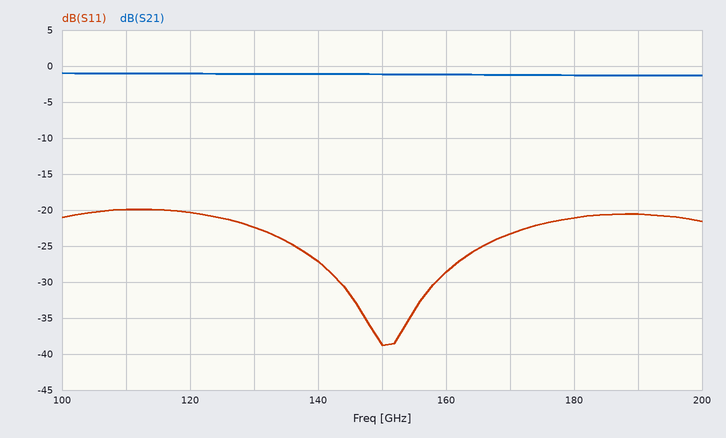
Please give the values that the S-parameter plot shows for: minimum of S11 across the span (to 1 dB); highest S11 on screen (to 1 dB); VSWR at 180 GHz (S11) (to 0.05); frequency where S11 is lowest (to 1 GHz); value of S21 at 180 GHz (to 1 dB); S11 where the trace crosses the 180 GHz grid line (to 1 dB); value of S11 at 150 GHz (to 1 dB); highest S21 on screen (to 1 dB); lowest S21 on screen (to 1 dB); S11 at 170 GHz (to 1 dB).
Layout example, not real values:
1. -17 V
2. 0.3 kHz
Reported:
1. -39 dB
2. -20 dB
3. 1.20
4. 150 GHz
5. -1 dB
6. -21 dB
7. -39 dB
8. -1 dB
9. -1 dB
10. -23 dB
